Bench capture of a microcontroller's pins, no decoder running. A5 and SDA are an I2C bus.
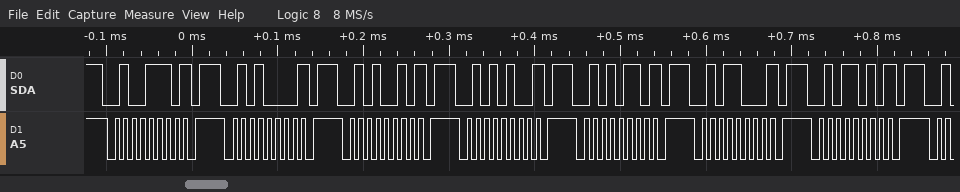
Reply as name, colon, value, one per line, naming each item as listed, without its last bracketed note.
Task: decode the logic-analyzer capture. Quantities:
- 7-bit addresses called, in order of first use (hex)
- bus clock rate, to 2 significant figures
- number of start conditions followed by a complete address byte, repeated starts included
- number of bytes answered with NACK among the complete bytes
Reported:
7-bit addresses called, in order of first use: 0x27 0x28 0x29 0x2A 0x2B 0x2C 0x2D
bus clock rate, to 2 significant figures: 100 kHz
number of start conditions followed by a complete address byte, repeated starts included: 7
number of bytes answered with NACK among the complete bytes: 7
